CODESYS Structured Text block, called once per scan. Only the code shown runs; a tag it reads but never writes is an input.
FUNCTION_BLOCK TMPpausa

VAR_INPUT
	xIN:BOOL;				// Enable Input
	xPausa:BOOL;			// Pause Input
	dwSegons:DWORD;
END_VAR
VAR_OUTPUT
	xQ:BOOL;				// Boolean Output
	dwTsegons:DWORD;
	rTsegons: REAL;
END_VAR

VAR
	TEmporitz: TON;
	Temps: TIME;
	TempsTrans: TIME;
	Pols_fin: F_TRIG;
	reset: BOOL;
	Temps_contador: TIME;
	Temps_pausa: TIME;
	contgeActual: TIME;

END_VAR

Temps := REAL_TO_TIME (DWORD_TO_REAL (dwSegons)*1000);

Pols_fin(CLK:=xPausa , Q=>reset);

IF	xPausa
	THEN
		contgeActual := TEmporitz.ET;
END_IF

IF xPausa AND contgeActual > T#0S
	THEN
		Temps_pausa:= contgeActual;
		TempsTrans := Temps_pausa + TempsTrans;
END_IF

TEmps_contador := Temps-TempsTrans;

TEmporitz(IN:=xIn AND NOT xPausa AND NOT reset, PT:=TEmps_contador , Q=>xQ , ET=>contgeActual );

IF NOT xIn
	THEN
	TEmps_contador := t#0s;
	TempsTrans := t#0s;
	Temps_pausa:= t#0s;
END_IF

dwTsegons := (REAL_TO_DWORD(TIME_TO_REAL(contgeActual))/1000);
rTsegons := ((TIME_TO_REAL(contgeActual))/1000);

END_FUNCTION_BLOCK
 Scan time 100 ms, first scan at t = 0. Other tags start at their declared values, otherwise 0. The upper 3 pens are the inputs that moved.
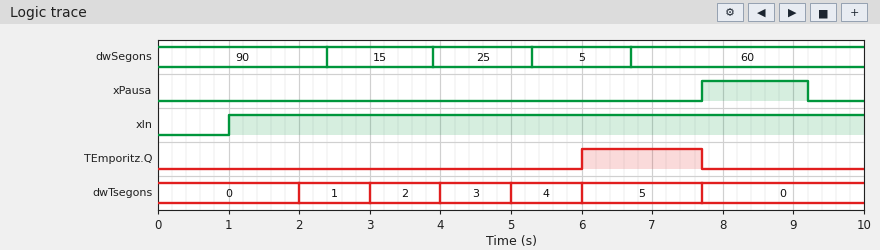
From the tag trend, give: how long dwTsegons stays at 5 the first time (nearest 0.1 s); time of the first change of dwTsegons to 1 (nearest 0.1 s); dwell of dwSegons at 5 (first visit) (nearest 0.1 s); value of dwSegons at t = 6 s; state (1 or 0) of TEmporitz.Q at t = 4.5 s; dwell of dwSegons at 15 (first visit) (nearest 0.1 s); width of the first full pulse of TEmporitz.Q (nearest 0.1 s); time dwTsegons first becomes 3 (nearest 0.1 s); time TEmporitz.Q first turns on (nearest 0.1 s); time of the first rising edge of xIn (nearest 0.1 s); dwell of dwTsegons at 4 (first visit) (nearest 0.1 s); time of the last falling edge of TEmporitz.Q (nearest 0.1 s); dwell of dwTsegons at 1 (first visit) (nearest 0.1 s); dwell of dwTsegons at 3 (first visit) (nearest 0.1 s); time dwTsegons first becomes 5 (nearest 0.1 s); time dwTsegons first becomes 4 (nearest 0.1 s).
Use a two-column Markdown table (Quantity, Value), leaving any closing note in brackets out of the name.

| Quantity | Value |
|---|---|
| how long dwTsegons stays at 5 the first time | 1.7 s |
| time of the first change of dwTsegons to 1 | 2.0 s |
| dwell of dwSegons at 5 (first visit) | 1.4 s |
| value of dwSegons at t = 6 s | 5 |
| state (1 or 0) of TEmporitz.Q at t = 4.5 s | 0 |
| dwell of dwSegons at 15 (first visit) | 1.5 s |
| width of the first full pulse of TEmporitz.Q | 1.7 s |
| time dwTsegons first becomes 3 | 4.0 s |
| time TEmporitz.Q first turns on | 6.0 s |
| time of the first rising edge of xIn | 1.0 s |
| dwell of dwTsegons at 4 (first visit) | 1.0 s |
| time of the last falling edge of TEmporitz.Q | 7.7 s |
| dwell of dwTsegons at 1 (first visit) | 1.0 s |
| dwell of dwTsegons at 3 (first visit) | 1.0 s |
| time dwTsegons first becomes 5 | 6.0 s |
| time dwTsegons first becomes 4 | 5.0 s |
